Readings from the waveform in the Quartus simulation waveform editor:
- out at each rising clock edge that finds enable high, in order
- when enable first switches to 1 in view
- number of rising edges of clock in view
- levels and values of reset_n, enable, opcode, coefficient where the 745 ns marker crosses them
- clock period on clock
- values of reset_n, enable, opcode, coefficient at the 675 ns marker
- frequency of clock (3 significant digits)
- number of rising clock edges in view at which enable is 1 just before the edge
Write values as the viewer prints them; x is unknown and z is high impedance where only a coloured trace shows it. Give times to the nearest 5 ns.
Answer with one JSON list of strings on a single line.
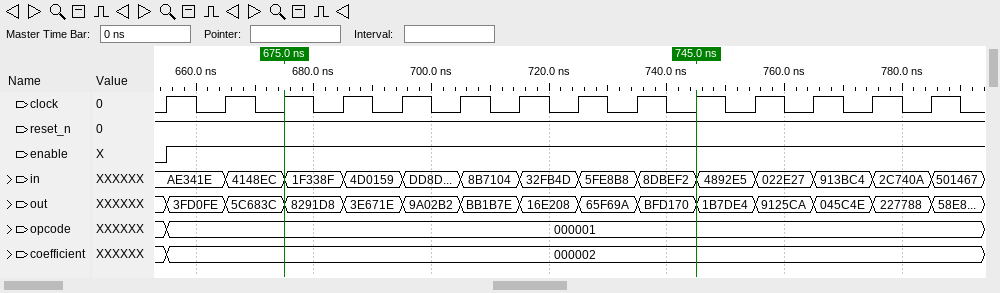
["3FD0FE, 5C683C, 8291D8, 3E671E, 9A02B2, BB1B7E, 16E208, 65F69A, BFD170, 1B7DE4, 9125CA, 045C4E, 227788", "655 ns", "14", "reset_n=1, enable=1, opcode=000001, coefficient=000002", "10 ns", "reset_n=1, enable=1, opcode=000001, coefficient=000002", "100 MHz", "13"]
